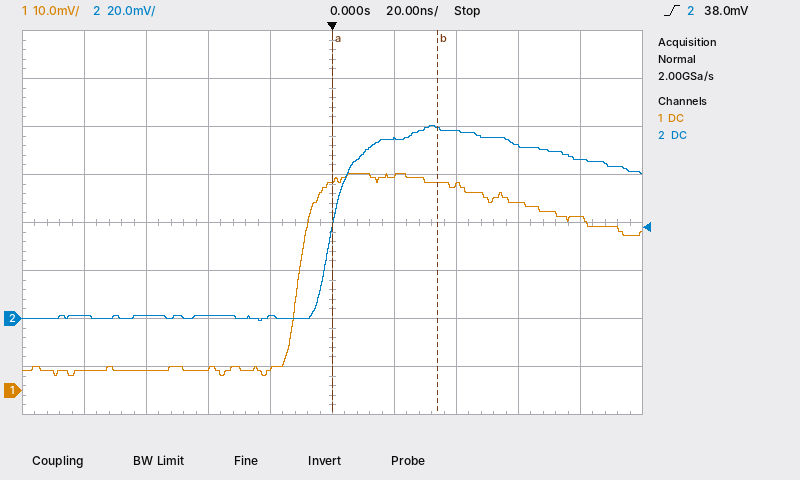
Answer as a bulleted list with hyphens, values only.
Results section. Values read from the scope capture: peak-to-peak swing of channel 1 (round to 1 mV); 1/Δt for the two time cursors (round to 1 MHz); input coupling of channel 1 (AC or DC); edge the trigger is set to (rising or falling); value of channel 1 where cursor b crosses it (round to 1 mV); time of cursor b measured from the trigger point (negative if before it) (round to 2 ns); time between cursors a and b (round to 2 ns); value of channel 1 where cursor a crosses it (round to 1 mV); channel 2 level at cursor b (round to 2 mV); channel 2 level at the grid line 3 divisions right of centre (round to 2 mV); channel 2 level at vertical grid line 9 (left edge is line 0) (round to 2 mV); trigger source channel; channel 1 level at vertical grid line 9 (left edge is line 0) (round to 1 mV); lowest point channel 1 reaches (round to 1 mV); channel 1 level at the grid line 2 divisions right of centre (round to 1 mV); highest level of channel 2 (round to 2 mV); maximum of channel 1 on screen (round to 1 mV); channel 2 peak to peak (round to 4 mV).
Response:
- 42 mV
- 29 MHz
- DC
- rising
- 43 mV
- +34 ns
- 34 ns
- 44 mV
- 80 mV
- 72 mV
- 66 mV
- channel 2
- 36 mV
- 3 mV
- 43 mV
- 80 mV
- 45 mV
- 80 mV
